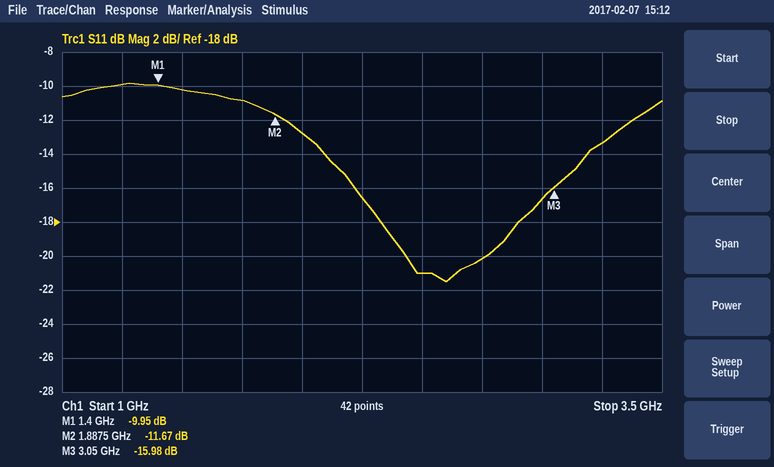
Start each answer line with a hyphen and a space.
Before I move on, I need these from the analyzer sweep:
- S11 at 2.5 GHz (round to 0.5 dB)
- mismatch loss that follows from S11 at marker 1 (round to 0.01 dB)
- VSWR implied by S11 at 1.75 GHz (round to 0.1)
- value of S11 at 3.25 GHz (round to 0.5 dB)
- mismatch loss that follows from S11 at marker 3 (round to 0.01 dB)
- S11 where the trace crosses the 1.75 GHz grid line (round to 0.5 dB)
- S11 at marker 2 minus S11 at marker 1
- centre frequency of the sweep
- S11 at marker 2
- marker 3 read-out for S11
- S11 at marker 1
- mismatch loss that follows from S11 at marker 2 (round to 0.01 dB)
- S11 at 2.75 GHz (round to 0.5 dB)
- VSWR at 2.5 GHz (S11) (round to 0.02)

- -21.0 dB
- 0.46 dB
- 1.8
- -13.5 dB
- 0.11 dB
- -11.0 dB
- -1.72 dB
- 2.25 GHz
- -11.67 dB
- -15.98 dB
- -9.95 dB
- 0.31 dB
- -20.0 dB
- 1.20
